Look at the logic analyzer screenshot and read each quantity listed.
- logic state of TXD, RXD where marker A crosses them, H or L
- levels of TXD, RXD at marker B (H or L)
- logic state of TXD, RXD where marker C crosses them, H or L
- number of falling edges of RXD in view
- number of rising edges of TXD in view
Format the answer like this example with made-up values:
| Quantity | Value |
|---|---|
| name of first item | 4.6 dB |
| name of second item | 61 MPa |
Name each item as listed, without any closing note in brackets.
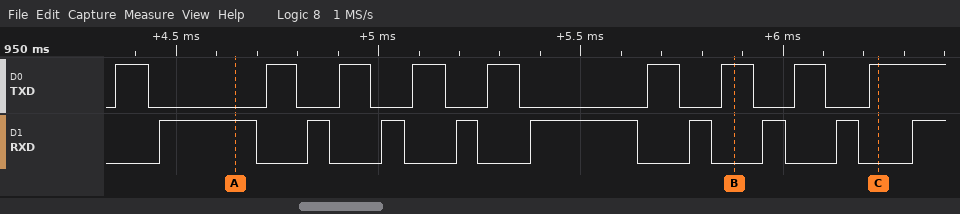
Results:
| Quantity | Value |
|---|---|
| logic state of TXD, RXD where marker A crosses them, H or L | TXD=L, RXD=H |
| levels of TXD, RXD at marker B | TXD=H, RXD=L |
| logic state of TXD, RXD where marker C crosses them, H or L | TXD=H, RXD=L |
| number of falling edges of RXD in view | 8 |
| number of rising edges of TXD in view | 9 |
